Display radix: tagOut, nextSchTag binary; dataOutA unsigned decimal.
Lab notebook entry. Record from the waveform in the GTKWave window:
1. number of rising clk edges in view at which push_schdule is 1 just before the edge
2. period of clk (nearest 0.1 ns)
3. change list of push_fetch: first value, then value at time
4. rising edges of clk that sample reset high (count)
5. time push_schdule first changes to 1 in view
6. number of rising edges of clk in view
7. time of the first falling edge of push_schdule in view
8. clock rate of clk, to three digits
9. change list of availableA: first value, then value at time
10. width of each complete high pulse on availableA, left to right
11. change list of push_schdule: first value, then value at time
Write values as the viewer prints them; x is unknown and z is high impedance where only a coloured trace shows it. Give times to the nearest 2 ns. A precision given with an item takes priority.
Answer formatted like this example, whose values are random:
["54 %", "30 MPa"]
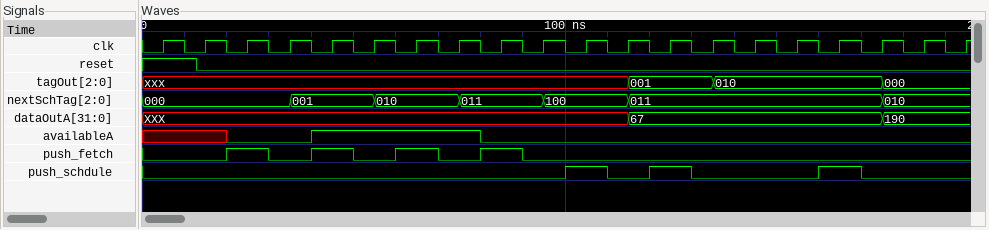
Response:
["3", "10 ns", "0, 1 at 20 ns, 0 at 30 ns, 1 at 40 ns, 0 at 50 ns, 1 at 60 ns, 0 at 70 ns, 1 at 80 ns, 0 at 90 ns", "1", "100 ns", "20", "110 ns", "100 MHz", "x, 0 at 20 ns, 1 at 40 ns, 0 at 80 ns", "40 ns", "0, 1 at 100 ns, 0 at 110 ns, 1 at 120 ns, 0 at 130 ns, 1 at 160 ns, 0 at 170 ns"]
